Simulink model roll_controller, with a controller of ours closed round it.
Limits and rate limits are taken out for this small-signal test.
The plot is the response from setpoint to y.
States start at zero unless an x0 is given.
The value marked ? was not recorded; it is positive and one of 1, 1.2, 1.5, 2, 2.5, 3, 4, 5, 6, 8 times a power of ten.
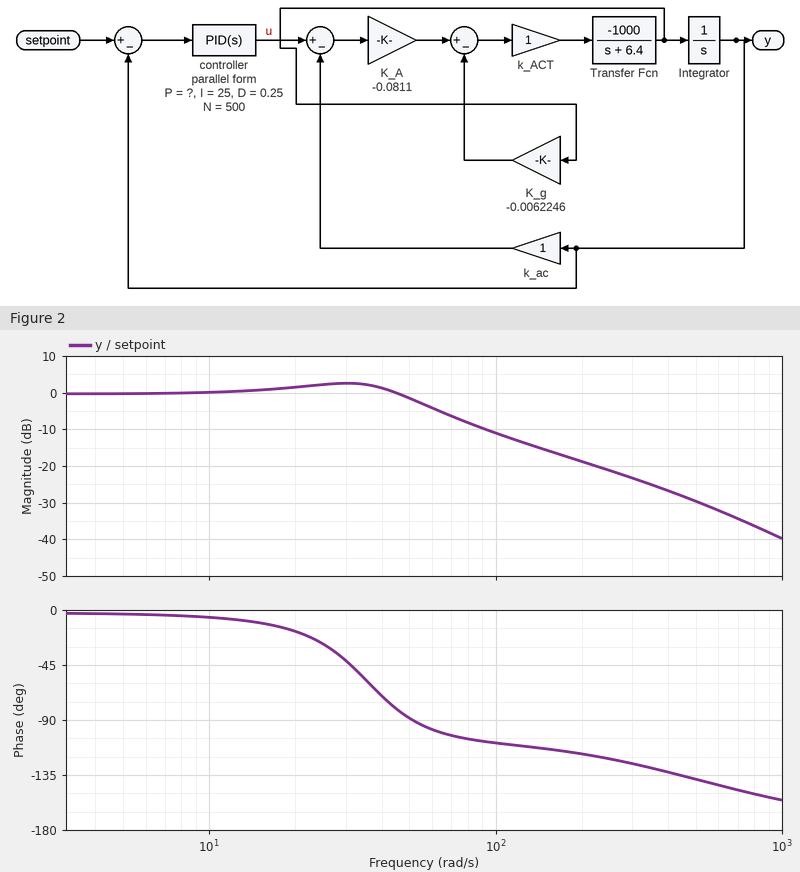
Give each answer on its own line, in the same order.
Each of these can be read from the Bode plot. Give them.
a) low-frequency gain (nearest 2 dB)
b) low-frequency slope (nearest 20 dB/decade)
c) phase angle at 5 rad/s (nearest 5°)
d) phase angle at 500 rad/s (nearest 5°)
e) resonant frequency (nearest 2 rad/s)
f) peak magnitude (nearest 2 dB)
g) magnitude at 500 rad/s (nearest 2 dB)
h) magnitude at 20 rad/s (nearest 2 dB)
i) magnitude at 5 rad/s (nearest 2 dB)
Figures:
0 dB
0 dB/decade
-5°
-140°
30 rad/s
2 dB
-30 dB
2 dB
0 dB
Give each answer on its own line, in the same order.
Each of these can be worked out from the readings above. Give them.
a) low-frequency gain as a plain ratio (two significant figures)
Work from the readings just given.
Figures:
1.0
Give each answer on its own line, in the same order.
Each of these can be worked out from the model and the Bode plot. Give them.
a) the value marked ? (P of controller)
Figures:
15
